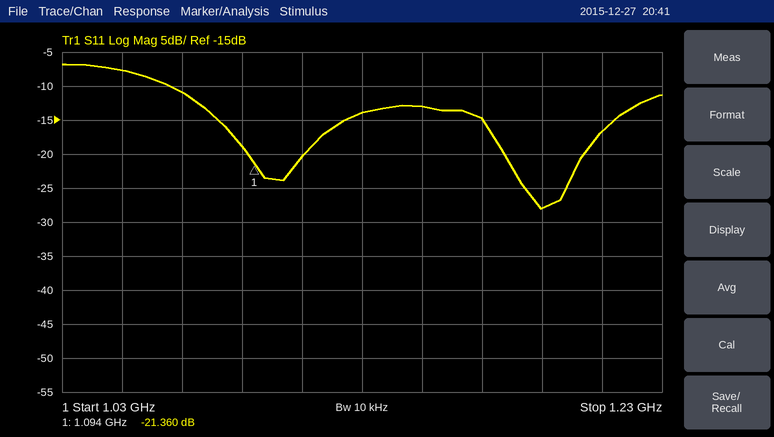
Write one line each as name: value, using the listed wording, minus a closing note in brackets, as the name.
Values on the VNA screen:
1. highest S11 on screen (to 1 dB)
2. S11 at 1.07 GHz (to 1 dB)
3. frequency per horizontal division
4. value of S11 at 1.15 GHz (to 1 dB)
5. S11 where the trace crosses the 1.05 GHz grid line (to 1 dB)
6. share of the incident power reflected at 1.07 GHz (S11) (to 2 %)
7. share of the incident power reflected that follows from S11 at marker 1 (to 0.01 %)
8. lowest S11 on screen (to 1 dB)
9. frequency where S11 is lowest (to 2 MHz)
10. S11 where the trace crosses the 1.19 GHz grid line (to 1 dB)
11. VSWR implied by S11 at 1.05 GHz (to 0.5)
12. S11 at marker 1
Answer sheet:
highest S11 on screen: -7 dB
S11 at 1.07 GHz: -11 dB
frequency per horizontal division: 20 MHz
value of S11 at 1.15 GHz: -13 dB
S11 where the trace crosses the 1.05 GHz grid line: -8 dB
share of the incident power reflected at 1.07 GHz (S11): 8 %
share of the incident power reflected that follows from S11 at marker 1: 0.73 %
lowest S11 on screen: -28 dB
frequency where S11 is lowest: 1.190 GHz
S11 where the trace crosses the 1.19 GHz grid line: -28 dB
VSWR implied by S11 at 1.05 GHz: 2.5
S11 at marker 1: -21.360 dB
